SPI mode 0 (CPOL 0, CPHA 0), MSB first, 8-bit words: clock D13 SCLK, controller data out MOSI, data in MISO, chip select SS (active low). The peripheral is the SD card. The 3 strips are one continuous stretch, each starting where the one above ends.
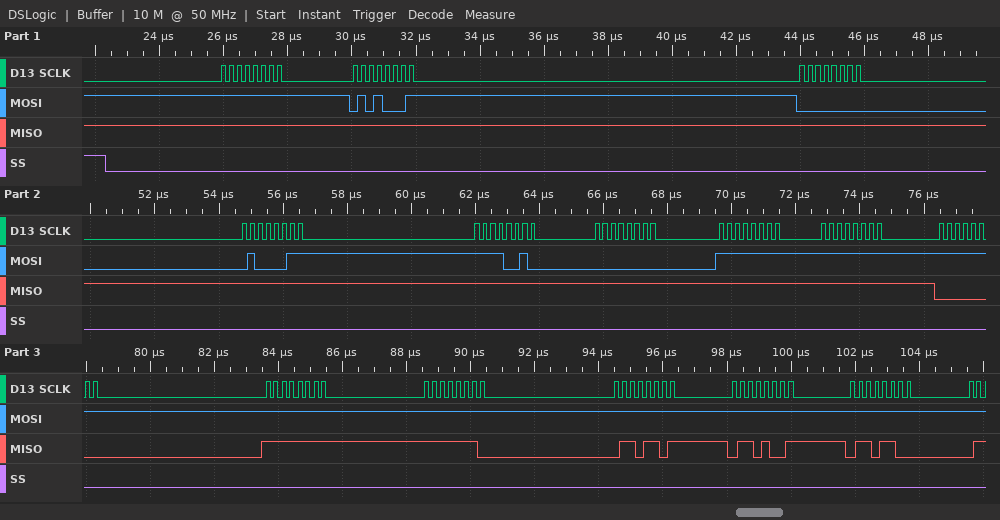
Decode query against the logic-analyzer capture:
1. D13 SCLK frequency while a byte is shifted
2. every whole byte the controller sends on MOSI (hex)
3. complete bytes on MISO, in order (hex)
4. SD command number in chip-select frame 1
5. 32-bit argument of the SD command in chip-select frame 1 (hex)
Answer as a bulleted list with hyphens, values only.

- 4 MHz
- FF 51 00 43 F2 00 FF FF FF FF FF FF FF FF
- FF FF FF FF FF FF FF FF 00 FF FE 6D 69 6C
- CMD17
- 0x0043F200
